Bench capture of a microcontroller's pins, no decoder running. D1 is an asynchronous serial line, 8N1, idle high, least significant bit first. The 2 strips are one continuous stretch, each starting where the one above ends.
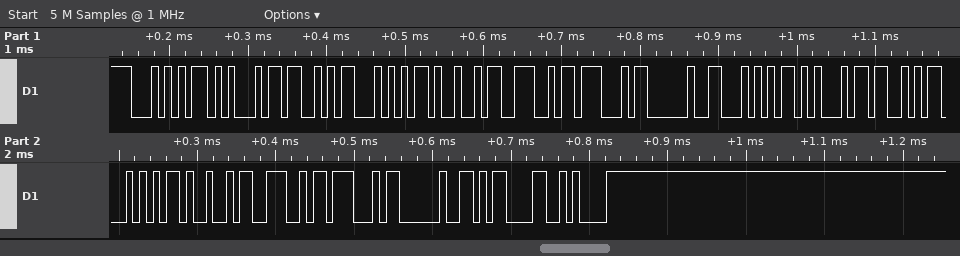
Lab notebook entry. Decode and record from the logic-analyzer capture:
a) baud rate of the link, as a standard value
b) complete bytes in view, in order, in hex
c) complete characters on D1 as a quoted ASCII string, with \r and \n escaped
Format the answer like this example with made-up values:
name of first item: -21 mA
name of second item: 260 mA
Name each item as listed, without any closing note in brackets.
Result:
baud rate of the link, as a standard value: 115200 baud
complete bytes in view, in order, in hex: 54 45 53 54 49 4E 47 20 54 45 53 54 49 4E 47 20 0D 0A
complete characters on D1 as a quoted ASCII string, with \r and \n escaped: "TESTING TESTING \r\n"
